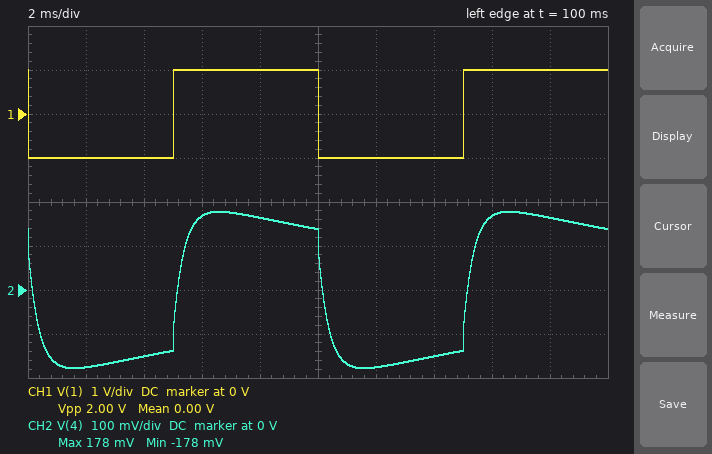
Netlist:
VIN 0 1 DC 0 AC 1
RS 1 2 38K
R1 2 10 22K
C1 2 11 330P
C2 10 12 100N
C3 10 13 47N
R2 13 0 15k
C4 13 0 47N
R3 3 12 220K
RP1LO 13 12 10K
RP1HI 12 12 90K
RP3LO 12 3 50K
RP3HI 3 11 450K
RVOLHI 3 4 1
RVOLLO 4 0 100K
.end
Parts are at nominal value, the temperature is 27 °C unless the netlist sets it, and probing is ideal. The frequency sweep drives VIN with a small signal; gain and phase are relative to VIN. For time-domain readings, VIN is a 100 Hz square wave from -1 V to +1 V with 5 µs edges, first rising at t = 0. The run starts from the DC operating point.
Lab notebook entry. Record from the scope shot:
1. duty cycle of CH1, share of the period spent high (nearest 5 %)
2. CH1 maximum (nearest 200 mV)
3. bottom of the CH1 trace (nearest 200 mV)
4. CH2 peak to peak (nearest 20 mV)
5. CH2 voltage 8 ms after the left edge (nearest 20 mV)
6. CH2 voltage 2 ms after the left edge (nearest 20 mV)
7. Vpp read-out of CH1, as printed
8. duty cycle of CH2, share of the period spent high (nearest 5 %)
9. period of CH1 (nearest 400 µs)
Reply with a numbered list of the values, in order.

1. 50 %
2. 1.0 V
3. -1.0 V
4. 360 mV
5. 160 mV
6. -180 mV
7. 2.00 V
8. 50 %
9. 10.0 ms
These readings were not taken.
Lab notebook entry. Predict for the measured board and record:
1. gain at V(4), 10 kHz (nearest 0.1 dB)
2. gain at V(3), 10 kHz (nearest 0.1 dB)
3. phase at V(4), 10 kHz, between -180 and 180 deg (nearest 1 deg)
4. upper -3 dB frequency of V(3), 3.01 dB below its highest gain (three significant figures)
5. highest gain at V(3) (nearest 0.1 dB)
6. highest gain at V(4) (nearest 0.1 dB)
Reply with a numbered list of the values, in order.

1. -32.9 dB
2. -32.9 dB
3. 165 deg
4. 437 Hz
5. -15.7 dB
6. -15.7 dB
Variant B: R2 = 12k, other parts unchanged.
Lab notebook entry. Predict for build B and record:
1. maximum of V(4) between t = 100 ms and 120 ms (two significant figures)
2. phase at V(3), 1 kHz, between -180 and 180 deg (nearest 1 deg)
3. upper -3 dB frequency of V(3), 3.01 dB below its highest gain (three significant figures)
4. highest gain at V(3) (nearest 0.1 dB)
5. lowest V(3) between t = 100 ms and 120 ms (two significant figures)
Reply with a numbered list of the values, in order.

1. 170 mV
2. 132 deg
3. 502 Hz
4. -16.5 dB
5. -170 mV
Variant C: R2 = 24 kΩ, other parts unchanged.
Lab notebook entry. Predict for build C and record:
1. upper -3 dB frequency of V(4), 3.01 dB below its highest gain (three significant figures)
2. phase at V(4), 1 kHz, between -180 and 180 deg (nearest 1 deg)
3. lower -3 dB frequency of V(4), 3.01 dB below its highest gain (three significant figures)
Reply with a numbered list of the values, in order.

1. 317 Hz
2. 128 deg
3. 11.6 Hz
